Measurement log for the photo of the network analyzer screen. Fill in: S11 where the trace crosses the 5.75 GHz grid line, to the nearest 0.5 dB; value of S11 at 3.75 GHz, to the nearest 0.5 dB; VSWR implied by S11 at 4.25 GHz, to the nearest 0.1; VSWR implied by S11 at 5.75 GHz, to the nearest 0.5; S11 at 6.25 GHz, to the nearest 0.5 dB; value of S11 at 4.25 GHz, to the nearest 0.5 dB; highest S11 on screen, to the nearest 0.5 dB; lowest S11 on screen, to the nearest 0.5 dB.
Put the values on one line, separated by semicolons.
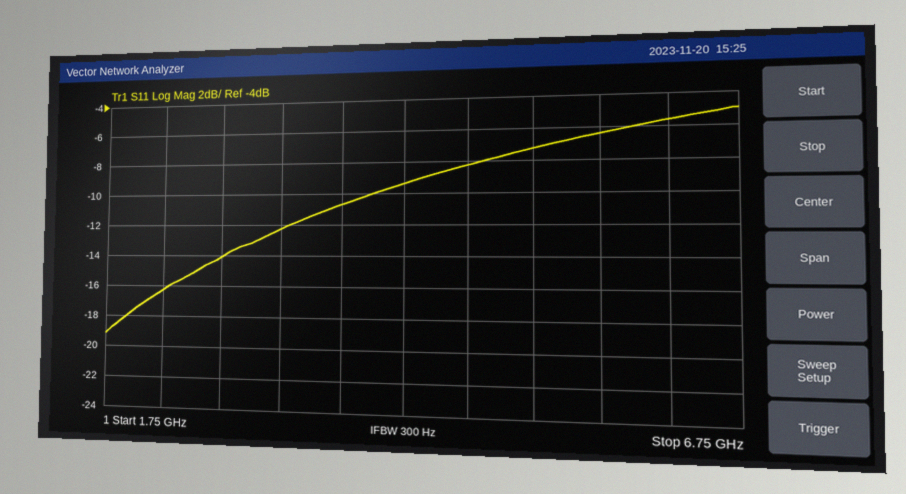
-6.5 dB; -10.5 dB; 2.0; 3.0; -5.5 dB; -9.5 dB; -5.0 dB; -19.0 dB
